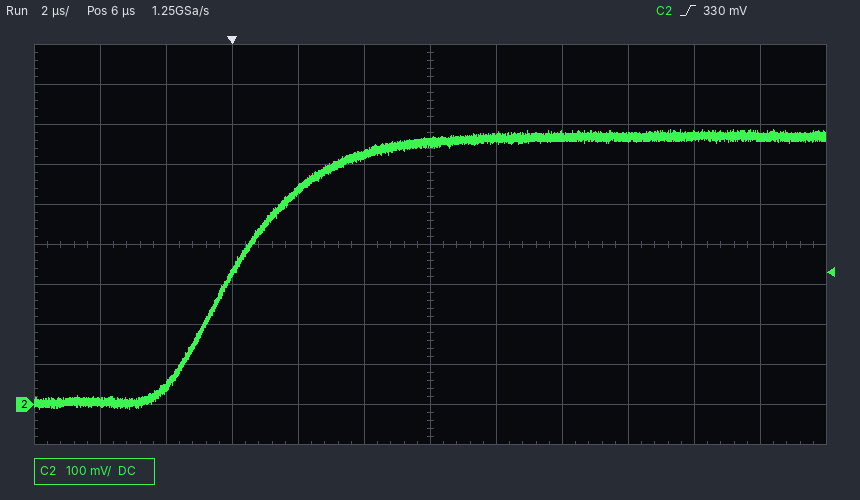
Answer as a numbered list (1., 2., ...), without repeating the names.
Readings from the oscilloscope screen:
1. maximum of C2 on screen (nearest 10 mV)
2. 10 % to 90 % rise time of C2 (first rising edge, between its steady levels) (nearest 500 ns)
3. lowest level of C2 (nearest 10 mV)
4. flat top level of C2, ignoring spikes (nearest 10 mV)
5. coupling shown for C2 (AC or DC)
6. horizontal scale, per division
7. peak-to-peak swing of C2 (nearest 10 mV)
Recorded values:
1. 690 mV
2. 5.0 µs
3. -10 mV
4. 670 mV
5. DC
6. 2 µs
7. 700 mV
